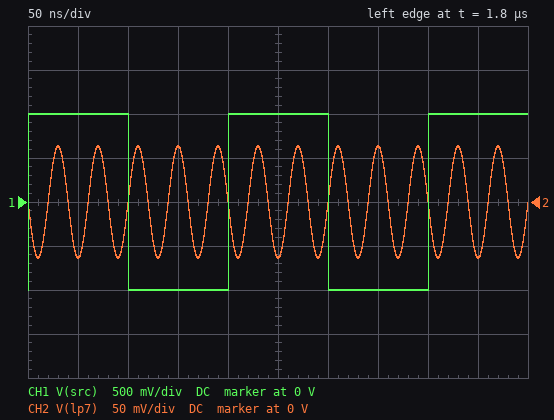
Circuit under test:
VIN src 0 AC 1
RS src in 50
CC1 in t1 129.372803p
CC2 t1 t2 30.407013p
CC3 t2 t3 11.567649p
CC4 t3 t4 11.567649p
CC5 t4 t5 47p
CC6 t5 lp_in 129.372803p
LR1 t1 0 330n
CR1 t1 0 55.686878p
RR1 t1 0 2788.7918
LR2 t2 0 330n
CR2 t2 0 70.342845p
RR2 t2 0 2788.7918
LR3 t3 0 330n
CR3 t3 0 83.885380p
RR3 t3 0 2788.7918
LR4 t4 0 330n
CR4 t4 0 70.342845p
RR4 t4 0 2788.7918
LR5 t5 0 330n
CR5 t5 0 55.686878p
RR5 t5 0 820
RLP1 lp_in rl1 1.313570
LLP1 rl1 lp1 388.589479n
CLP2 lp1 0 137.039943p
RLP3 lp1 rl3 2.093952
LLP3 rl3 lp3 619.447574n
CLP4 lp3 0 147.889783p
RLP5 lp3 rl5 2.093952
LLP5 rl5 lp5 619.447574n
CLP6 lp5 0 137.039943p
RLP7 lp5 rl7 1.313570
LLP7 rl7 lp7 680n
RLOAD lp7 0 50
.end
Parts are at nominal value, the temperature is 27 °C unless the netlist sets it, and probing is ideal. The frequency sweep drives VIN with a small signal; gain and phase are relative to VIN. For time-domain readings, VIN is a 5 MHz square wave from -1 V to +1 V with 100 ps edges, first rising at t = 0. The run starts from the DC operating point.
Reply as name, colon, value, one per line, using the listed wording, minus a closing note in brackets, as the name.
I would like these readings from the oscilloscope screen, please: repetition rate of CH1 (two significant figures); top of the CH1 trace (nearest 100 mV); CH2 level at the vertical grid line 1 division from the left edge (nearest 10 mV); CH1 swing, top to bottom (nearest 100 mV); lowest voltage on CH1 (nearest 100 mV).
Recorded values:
repetition rate of CH1: 5.0 MHz
top of the CH1 trace: 1.0 V
CH2 level at the vertical grid line 1 division from the left edge: -60 mV
CH1 swing, top to bottom: 2.0 V
lowest voltage on CH1: -1.0 V
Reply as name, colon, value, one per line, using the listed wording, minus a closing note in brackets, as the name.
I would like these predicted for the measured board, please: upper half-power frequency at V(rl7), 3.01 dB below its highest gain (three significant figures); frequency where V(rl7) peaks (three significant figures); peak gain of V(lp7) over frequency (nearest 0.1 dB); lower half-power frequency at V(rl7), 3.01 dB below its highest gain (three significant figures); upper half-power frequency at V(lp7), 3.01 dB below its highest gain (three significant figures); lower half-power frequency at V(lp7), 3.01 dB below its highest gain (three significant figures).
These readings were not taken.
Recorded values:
upper half-power frequency at V(rl7), 3.01 dB below its highest gain: 28.6 MHz
frequency where V(rl7) peaks: 26.1 MHz
peak gain of V(lp7) over frequency: -10.9 dB
lower half-power frequency at V(rl7), 3.01 dB below its highest gain: 24.8 MHz
upper half-power frequency at V(lp7), 3.01 dB below its highest gain: 28.3 MHz
lower half-power frequency at V(lp7), 3.01 dB below its highest gain: 24.8 MHz
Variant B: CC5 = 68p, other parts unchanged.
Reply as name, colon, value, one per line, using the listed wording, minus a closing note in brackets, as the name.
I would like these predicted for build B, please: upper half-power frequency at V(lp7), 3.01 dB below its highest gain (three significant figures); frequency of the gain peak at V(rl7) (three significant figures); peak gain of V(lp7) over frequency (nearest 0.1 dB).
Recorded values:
upper half-power frequency at V(lp7), 3.01 dB below its highest gain: 27.5 MHz
frequency of the gain peak at V(rl7): 25.9 MHz
peak gain of V(lp7) over frequency: -11.3 dB
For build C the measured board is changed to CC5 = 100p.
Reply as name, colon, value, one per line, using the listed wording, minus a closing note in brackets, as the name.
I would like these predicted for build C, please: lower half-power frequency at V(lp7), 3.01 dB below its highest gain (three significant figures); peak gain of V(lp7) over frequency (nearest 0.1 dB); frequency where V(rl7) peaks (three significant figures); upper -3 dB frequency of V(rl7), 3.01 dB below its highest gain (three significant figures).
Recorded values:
lower half-power frequency at V(lp7), 3.01 dB below its highest gain: 24.8 MHz
peak gain of V(lp7) over frequency: -11.9 dB
frequency where V(rl7) peaks: 25.8 MHz
upper -3 dB frequency of V(rl7), 3.01 dB below its highest gain: 28.3 MHz
